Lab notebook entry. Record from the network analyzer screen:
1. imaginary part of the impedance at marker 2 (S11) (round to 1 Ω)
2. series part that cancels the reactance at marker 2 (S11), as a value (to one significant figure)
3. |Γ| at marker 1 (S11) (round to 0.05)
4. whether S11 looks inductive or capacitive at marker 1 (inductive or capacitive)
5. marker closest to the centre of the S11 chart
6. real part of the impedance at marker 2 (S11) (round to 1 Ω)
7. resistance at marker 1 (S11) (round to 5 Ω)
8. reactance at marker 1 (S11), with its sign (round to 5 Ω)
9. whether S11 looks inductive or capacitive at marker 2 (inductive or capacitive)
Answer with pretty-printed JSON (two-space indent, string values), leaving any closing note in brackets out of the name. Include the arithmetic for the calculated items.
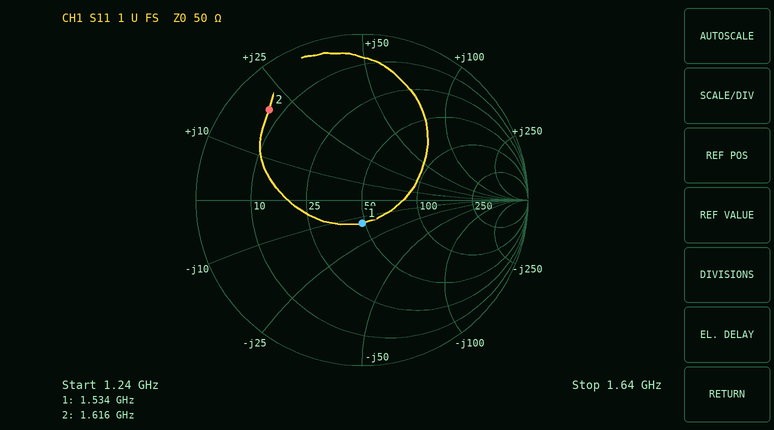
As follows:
{
  "imaginary part of the impedance at marker 2 (S11)": "+20 Ω",
  "series part that cancels the reactance at marker 2 (S11), as a value": "C = 1/(2π × 1.616 GHz × 20 Ω) ≈ 5 pF",
  "|Γ| at marker 1 (S11)": "0.15",
  "whether S11 looks inductive or capacitive at marker 1": "capacitive",
  "marker closest to the centre of the S11 chart": "marker 1",
  "real part of the impedance at marker 2 (S11)": "7 Ω",
  "resistance at marker 1 (S11)": "50 Ω",
  "reactance at marker 1 (S11), with its sign": "-15 Ω",
  "whether S11 looks inductive or capacitive at marker 2": "inductive"
}
